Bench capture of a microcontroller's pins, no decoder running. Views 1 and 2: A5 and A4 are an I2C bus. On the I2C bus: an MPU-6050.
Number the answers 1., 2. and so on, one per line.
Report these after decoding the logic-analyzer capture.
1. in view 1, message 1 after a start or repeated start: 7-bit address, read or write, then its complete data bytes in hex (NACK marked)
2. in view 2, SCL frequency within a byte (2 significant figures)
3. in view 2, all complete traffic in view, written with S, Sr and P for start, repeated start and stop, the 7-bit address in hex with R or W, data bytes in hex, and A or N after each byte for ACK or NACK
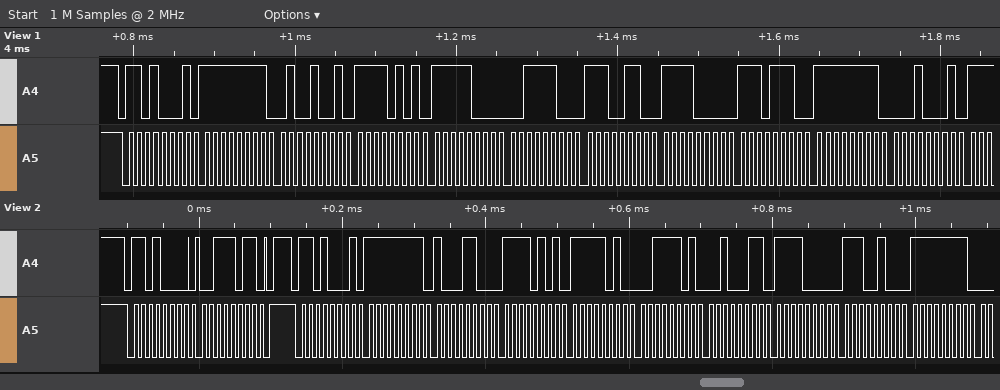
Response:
1. 0x68 read: FF 49 F5 F8 3C E6 F0 EE FF 11
2. 100 kHz
3. S 68W A 3B A P S 68R A FF A 8C A F5 A FA A 3D A 23 A F0 A E4 A FF A
